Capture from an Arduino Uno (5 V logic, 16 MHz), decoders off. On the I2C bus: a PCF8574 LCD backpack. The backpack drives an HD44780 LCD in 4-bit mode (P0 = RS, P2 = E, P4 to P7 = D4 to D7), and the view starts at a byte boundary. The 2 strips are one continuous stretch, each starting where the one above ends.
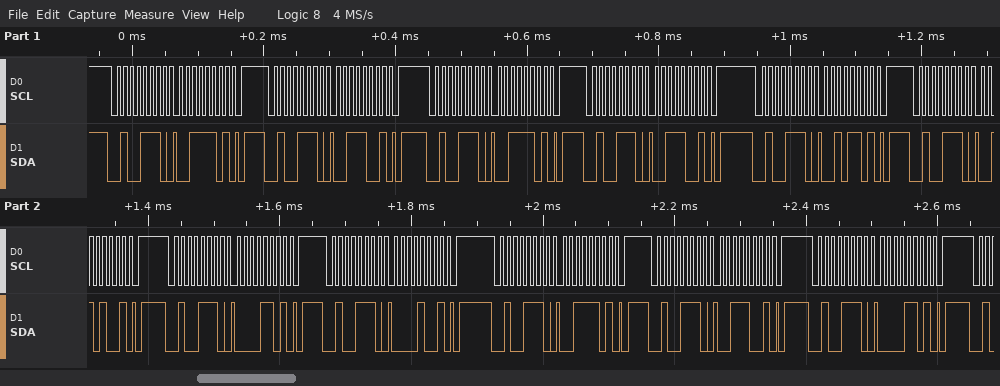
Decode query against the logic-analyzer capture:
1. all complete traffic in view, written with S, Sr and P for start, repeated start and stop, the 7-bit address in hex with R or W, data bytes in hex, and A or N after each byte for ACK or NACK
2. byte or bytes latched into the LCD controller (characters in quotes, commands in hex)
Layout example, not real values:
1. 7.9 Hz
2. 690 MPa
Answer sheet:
1. S 27W A 3D A P S 27W A 39 A P S 27W A 3D A P S 27W A 39 A P S 27W A 2D A P S 27W A 29 A P S 27W A 0D A P S 27W A 09 A P S 27W A 3D A P S 27W A 39 A P S 27W A 0D A P
2. '3' ' '
